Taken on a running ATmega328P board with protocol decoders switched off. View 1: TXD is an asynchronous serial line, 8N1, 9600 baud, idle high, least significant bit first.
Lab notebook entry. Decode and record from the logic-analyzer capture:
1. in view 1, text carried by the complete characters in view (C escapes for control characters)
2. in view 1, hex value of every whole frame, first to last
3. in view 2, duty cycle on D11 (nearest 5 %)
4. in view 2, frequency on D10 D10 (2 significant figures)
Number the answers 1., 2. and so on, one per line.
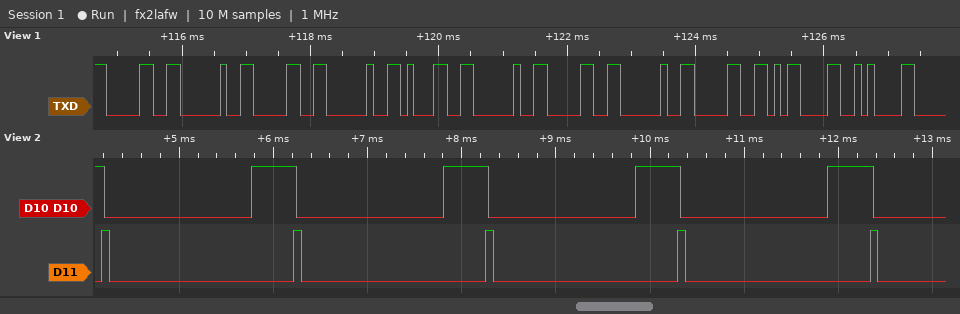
1. "0 0 1 0 0\r\n"
2. 30 20 30 20 31 20 30 20 30 0D 0A
3. 5 %
4. 490 Hz
